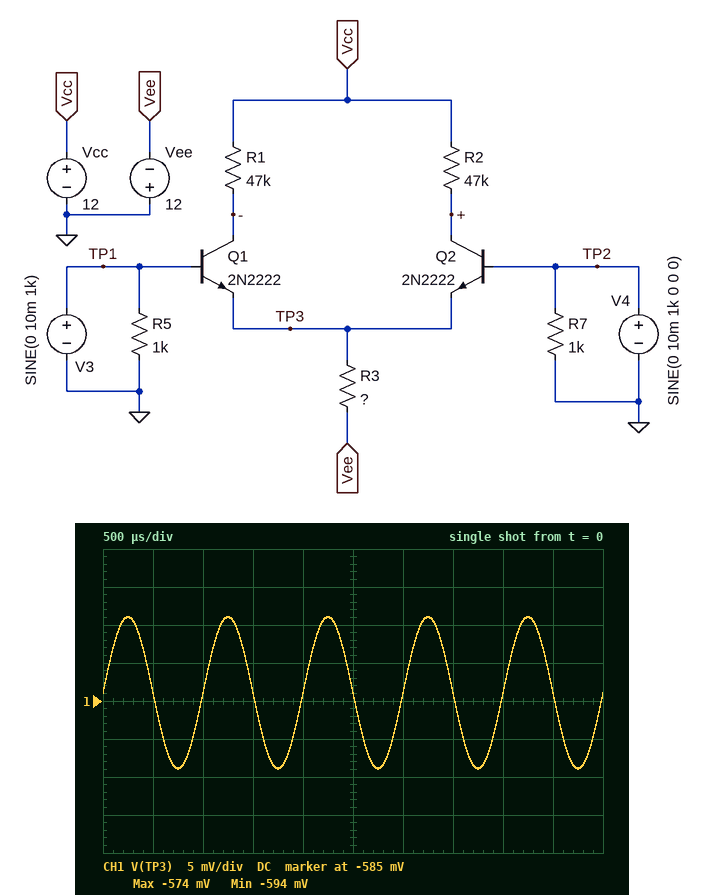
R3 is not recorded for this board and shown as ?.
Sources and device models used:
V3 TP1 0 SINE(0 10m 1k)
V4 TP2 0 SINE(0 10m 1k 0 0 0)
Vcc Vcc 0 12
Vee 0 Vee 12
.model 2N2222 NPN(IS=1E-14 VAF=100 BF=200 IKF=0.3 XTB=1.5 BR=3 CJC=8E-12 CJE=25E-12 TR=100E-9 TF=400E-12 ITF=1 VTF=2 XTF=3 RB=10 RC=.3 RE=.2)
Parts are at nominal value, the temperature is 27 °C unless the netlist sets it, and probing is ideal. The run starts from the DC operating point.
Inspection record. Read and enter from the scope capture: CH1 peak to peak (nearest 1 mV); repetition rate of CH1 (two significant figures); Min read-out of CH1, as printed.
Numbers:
20 mV
1.0 kHz
-594 mV
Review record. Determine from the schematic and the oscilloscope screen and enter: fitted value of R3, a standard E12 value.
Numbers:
82 kΩ
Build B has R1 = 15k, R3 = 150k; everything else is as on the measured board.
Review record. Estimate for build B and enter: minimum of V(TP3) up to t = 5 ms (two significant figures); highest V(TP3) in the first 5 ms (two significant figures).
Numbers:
-580 mV
-560 mV
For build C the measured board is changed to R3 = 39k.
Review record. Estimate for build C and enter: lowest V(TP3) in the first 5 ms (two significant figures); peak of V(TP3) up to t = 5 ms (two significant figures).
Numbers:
-610 mV
-590 mV
